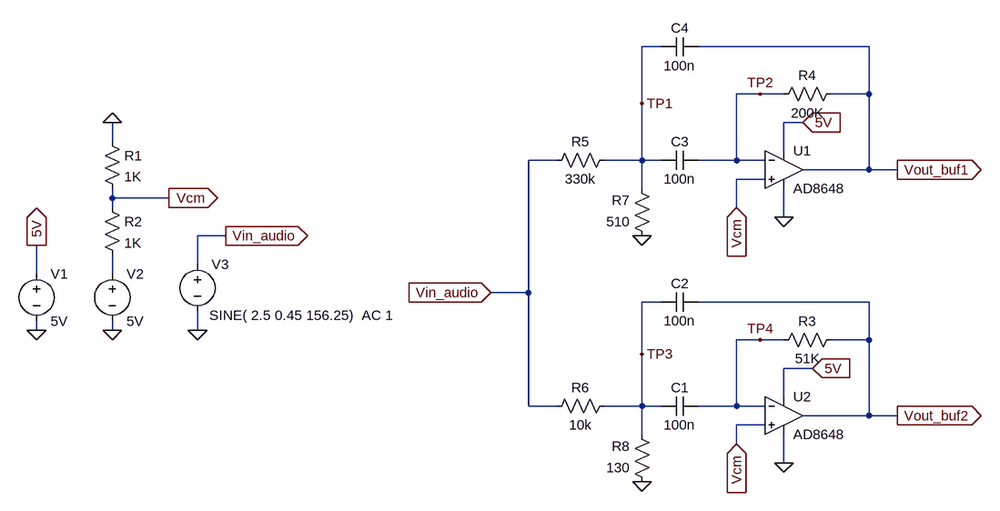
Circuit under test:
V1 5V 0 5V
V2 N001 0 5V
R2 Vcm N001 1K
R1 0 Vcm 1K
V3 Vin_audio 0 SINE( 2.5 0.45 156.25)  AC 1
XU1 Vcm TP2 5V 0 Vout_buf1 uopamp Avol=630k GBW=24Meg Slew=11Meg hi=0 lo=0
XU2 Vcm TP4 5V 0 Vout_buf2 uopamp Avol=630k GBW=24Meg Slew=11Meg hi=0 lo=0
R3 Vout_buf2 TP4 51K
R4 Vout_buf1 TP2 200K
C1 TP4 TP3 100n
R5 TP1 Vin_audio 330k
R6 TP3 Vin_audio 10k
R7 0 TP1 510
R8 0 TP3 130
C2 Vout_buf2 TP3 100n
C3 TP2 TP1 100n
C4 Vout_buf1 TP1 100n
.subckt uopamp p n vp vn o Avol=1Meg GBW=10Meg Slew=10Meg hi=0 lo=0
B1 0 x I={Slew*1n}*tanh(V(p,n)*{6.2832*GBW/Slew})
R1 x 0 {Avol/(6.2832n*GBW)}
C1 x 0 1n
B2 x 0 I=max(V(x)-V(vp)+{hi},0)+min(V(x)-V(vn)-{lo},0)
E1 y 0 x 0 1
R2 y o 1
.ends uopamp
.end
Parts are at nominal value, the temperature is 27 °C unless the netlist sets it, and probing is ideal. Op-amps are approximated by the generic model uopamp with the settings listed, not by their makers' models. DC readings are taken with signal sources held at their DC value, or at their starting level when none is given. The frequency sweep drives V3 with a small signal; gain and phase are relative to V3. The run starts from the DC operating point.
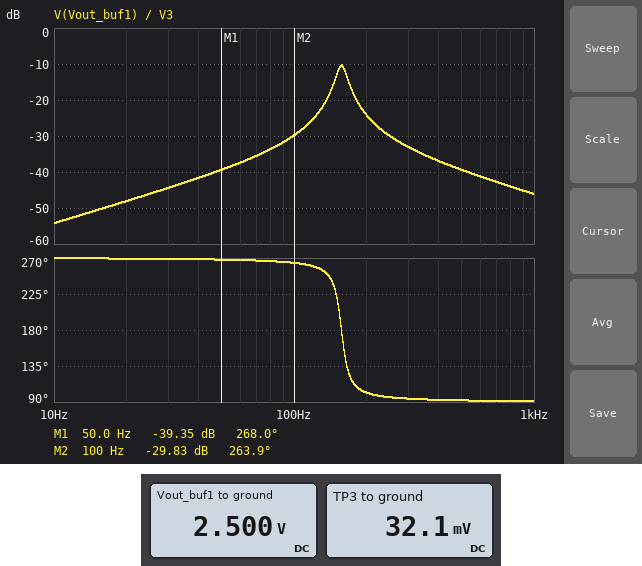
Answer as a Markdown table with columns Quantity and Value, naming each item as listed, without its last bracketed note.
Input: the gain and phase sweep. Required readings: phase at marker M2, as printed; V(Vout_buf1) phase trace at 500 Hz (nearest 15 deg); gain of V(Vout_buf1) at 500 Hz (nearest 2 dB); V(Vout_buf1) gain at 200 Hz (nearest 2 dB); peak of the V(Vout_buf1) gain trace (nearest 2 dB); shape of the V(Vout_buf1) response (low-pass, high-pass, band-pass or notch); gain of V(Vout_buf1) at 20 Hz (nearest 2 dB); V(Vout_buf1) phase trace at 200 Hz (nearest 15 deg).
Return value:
| Quantity | Value |
|---|---|
| phase at marker M2, as printed | 263.9 deg |
| V(Vout_buf1) phase trace at 500 Hz | 90 deg |
| gain of V(Vout_buf1) at 500 Hz | -40 dB |
| V(Vout_buf1) gain at 200 Hz | -24 dB |
| peak of the V(Vout_buf1) gain trace | -10 dB |
| shape of the V(Vout_buf1) response | band-pass |
| gain of V(Vout_buf1) at 20 Hz | -48 dB |
| V(Vout_buf1) phase trace at 200 Hz | 105 deg |
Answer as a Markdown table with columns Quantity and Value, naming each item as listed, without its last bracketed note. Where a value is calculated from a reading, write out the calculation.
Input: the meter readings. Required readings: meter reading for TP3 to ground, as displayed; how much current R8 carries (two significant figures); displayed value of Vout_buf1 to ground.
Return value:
| Quantity | Value |
|---|---|
| meter reading for TP3 to ground, as displayed | 32.1 mV |
| how much current R8 carries | (32.1 mV) / 130 Ω = 250 µA |
| displayed value of Vout_buf1 to ground | 2.500 V |
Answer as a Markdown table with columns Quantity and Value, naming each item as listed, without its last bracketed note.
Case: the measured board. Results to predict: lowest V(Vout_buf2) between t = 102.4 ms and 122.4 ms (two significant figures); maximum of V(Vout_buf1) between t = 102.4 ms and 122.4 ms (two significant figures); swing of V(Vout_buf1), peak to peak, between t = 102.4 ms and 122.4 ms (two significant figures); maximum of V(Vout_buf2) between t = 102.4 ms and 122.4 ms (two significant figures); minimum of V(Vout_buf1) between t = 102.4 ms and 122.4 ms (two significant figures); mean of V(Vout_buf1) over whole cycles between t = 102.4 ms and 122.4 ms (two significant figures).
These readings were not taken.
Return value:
| Quantity | Value |
|---|---|
| lowest V(Vout_buf2) between t = 102.4 ms and 122.4 ms | 2.5 V |
| maximum of V(Vout_buf1) between t = 102.4 ms and 122.4 ms | 2.6 V |
| swing of V(Vout_buf1), peak to peak, between t = 102.4 ms and 122.4 ms | 270 mV |
| maximum of V(Vout_buf2) between t = 102.4 ms and 122.4 ms | 2.5 V |
| minimum of V(Vout_buf1) between t = 102.4 ms and 122.4 ms | 2.4 V |
| mean of V(Vout_buf1) over whole cycles between t = 102.4 ms and 122.4 ms | 2.5 V |
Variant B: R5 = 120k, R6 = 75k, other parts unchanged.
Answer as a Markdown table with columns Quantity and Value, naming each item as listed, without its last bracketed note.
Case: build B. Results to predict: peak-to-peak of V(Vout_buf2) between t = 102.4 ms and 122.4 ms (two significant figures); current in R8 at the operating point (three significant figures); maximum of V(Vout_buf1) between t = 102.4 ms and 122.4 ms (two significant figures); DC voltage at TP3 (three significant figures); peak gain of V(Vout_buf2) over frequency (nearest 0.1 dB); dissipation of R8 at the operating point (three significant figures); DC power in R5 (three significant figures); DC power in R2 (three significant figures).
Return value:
| Quantity | Value |
|---|---|
| peak-to-peak of V(Vout_buf2) between t = 102.4 ms and 122.4 ms | 8.3 mV |
| current in R8 at the operating point | 33.3 µA |
| maximum of V(Vout_buf1) between t = 102.4 ms and 122.4 ms | 2.9 V |
| DC voltage at TP3 | 4.33 mV |
| peak gain of V(Vout_buf2) over frequency | -9.4 dB |
| dissipation of R8 at the operating point | 144 nW |
| DC power in R5 | 51.6 µW |
| DC power in R2 | 6.25 mW |
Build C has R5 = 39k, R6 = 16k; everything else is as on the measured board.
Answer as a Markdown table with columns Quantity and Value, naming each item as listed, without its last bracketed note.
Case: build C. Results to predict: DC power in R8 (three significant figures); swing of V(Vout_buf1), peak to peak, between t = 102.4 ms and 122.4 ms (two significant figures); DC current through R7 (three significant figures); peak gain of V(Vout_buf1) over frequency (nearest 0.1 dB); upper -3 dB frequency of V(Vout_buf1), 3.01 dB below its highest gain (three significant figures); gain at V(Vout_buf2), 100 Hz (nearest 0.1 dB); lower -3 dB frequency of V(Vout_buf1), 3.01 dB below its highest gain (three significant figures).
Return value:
| Quantity | Value |
|---|---|
| DC power in R8 | 3.12 µW |
| swing of V(Vout_buf1), peak to peak, between t = 102.4 ms and 122.4 ms | 2.2 V |
| DC current through R7 | 63.3 µA |
| peak gain of V(Vout_buf1) over frequency | 8.2 dB |
| upper -3 dB frequency of V(Vout_buf1), 3.01 dB below its highest gain | 167 Hz |
| gain at V(Vout_buf2), 100 Hz | -31.5 dB |
| lower -3 dB frequency of V(Vout_buf1), 3.01 dB below its highest gain | 151 Hz |
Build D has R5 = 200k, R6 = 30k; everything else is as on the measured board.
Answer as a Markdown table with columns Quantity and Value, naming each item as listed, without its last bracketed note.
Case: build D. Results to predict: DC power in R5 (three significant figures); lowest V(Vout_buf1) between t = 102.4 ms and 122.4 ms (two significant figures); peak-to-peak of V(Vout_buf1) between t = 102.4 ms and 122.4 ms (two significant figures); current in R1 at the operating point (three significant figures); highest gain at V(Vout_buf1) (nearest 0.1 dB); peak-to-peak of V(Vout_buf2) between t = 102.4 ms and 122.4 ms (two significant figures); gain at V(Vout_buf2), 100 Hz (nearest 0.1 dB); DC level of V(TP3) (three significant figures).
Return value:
| Quantity | Value |
|---|---|
| DC power in R5 | 31.1 µW |
| lowest V(Vout_buf1) between t = 102.4 ms and 122.4 ms | 2.3 V |
| peak-to-peak of V(Vout_buf1) between t = 102.4 ms and 122.4 ms | 440 mV |
| current in R1 at the operating point | 2.50 mA |
| highest gain at V(Vout_buf1) | -6.0 dB |
| peak-to-peak of V(Vout_buf2) between t = 102.4 ms and 122.4 ms | 21 mV |
| gain at V(Vout_buf2), 100 Hz | -37.0 dB |
| DC level of V(TP3) | 10.8 mV |
